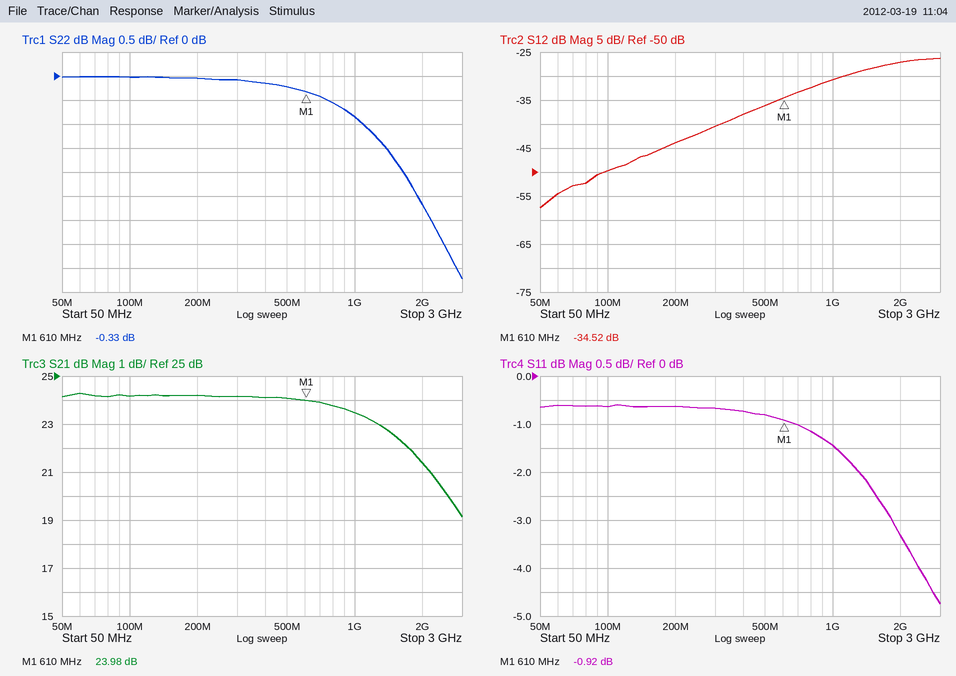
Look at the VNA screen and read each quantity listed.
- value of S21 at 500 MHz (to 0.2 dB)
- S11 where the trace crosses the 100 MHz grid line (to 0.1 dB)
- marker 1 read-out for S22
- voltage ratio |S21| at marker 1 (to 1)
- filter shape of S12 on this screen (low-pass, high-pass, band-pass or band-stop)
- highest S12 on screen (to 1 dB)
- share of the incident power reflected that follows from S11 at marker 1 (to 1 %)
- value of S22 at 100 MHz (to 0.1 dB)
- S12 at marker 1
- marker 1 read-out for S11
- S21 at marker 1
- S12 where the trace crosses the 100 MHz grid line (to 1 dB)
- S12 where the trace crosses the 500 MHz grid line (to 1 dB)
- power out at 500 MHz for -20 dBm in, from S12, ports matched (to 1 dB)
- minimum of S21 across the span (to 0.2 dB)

24.0 dB
-0.6 dB
-0.33 dB
16
high-pass
-26 dB
81 %
0.0 dB
-34.52 dB
-0.92 dB
23.98 dB
-50 dB
-36 dB
-56 dBm
19.2 dB
